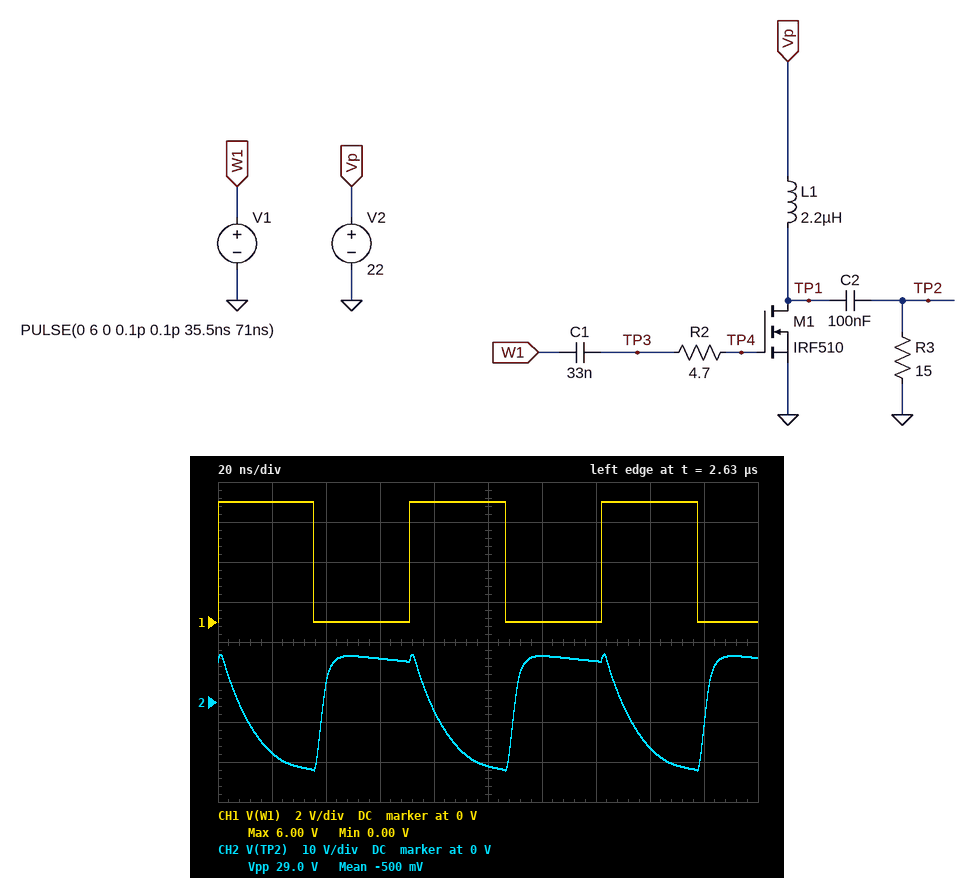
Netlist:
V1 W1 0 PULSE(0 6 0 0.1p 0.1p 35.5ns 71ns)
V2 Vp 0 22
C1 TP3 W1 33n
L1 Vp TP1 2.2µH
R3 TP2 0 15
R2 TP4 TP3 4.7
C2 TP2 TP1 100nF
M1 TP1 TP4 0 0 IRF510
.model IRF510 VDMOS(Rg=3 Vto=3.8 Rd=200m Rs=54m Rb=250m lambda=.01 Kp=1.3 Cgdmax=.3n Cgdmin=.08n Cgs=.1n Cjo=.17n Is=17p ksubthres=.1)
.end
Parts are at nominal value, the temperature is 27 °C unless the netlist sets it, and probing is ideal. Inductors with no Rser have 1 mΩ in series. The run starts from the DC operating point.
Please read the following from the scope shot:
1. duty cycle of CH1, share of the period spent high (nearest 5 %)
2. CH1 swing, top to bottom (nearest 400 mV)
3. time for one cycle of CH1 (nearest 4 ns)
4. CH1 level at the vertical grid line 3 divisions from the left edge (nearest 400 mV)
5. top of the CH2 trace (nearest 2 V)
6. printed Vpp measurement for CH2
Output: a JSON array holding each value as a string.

["50 %", "6.0 V", "72 ns", "0 V", "12 V", "29.0 V"]
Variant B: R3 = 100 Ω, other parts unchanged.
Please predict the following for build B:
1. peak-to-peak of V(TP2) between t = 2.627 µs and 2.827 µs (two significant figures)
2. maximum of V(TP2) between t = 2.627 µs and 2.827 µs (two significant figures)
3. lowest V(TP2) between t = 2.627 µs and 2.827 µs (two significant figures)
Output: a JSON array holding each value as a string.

["44 V", "22 V", "-22 V"]
